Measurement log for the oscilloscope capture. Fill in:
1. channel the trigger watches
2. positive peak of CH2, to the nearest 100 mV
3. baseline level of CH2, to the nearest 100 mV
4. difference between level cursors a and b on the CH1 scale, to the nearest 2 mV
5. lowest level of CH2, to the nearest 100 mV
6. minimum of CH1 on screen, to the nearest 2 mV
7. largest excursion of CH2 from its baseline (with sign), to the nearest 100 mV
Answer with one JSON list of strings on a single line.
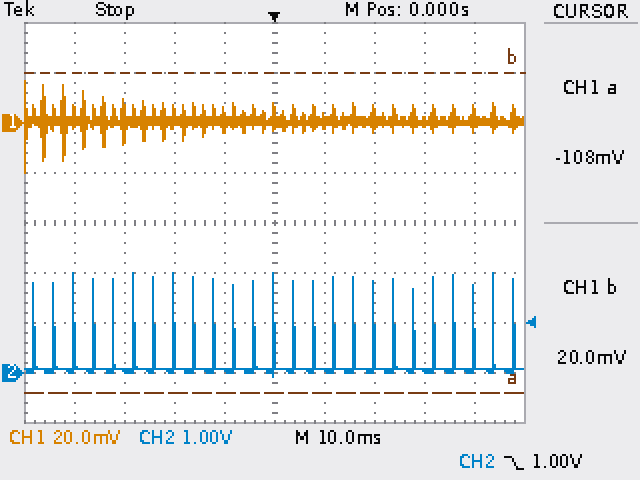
["CH2", "2.0 V", "100 mV", "128 mV", "-100 mV", "-20 mV", "+1.9 V"]
